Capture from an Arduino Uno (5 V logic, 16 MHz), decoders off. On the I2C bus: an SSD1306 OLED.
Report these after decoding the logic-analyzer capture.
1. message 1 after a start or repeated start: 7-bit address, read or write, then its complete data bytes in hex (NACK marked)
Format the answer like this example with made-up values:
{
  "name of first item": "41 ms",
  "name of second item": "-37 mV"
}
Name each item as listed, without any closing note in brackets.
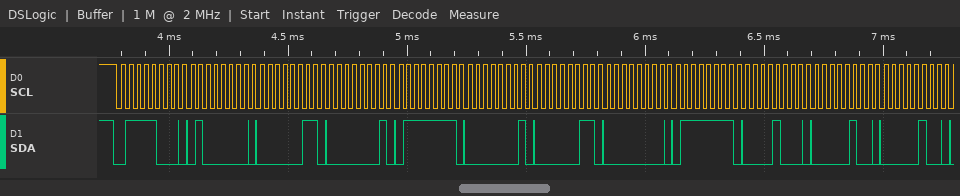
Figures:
{
  "message 1 after a start or repeated start: 7-bit address, read or write, then its complete data bytes in hex": "0x3C write: 40 03 01 7F 01 03 00 7F 08 04 04"
}
